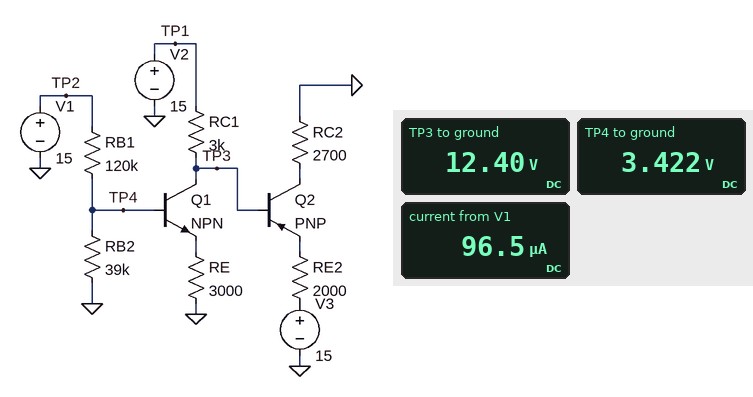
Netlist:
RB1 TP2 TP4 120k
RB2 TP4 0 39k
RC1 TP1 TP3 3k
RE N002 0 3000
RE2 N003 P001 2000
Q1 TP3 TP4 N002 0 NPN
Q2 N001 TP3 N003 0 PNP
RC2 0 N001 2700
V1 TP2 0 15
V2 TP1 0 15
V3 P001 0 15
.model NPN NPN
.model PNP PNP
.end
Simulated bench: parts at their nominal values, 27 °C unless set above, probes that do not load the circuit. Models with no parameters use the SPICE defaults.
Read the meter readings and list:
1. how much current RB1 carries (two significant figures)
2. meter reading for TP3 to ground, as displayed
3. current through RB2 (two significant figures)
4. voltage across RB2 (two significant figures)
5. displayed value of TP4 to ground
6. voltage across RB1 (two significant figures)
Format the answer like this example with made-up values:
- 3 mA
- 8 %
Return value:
- 96 µA
- 12.40 V
- 88 µA
- 3.4 V
- 3.422 V
- 12 V
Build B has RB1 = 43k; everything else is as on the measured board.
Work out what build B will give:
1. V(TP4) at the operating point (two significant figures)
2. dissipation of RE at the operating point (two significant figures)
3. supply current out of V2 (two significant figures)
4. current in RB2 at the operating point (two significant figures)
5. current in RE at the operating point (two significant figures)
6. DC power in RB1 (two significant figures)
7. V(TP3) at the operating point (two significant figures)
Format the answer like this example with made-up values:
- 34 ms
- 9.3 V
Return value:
- 6.7 V
- 12 mW
- 1.9 mA
- 170 µA
- 2.0 mA
- 1.6 mW
- 9.2 V
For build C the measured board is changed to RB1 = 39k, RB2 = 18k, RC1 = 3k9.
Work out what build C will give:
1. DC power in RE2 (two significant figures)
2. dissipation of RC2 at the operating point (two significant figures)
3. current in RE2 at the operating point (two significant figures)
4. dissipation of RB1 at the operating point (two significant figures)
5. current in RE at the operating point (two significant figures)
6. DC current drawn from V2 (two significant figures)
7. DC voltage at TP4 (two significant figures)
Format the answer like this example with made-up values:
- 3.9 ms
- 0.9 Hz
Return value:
- 8.1 mW
- 11 mW
- 2.0 mA
- 2.8 mW
- 1.3 mA
- 1.2 mA
- 4.6 V
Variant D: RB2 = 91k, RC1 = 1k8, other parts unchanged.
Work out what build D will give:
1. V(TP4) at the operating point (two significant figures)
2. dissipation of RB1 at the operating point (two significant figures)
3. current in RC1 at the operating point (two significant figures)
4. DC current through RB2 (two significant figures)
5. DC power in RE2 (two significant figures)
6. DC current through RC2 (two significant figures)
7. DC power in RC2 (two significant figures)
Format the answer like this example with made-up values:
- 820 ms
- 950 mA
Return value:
- 5.6 V
- 730 µW
- 1.6 mA
- 62 µA
- 2.2 mW
- 1.0 mA
- 2.9 mW
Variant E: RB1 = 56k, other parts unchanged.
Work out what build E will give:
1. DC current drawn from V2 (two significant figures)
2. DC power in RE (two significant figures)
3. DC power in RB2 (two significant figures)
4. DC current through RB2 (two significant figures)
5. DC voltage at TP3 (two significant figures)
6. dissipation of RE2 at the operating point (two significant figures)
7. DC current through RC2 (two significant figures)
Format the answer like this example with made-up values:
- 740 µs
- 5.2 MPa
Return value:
- 1.6 mA
- 8.3 mW
- 860 µW
- 150 µA
- 10 V
- 8.4 mW
- 2.0 mA
